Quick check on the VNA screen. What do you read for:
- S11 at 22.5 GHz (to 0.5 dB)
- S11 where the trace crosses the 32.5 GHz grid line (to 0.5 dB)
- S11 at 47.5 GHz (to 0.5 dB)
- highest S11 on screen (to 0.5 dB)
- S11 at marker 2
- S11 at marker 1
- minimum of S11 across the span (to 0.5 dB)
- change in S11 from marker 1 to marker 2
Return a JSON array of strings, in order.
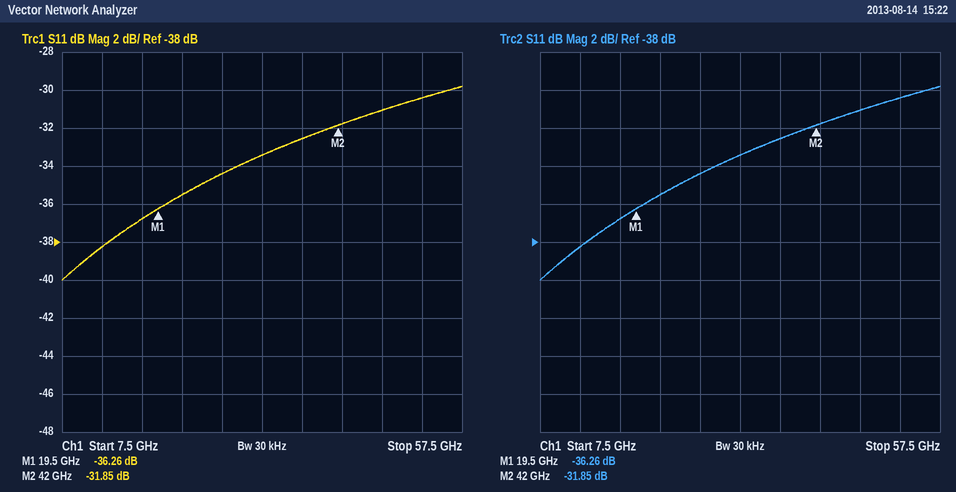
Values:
["-35.5 dB", "-33.5 dB", "-31.0 dB", "-30.0 dB", "-31.85 dB", "-36.26 dB", "-40.0 dB", "4.41 dB"]
